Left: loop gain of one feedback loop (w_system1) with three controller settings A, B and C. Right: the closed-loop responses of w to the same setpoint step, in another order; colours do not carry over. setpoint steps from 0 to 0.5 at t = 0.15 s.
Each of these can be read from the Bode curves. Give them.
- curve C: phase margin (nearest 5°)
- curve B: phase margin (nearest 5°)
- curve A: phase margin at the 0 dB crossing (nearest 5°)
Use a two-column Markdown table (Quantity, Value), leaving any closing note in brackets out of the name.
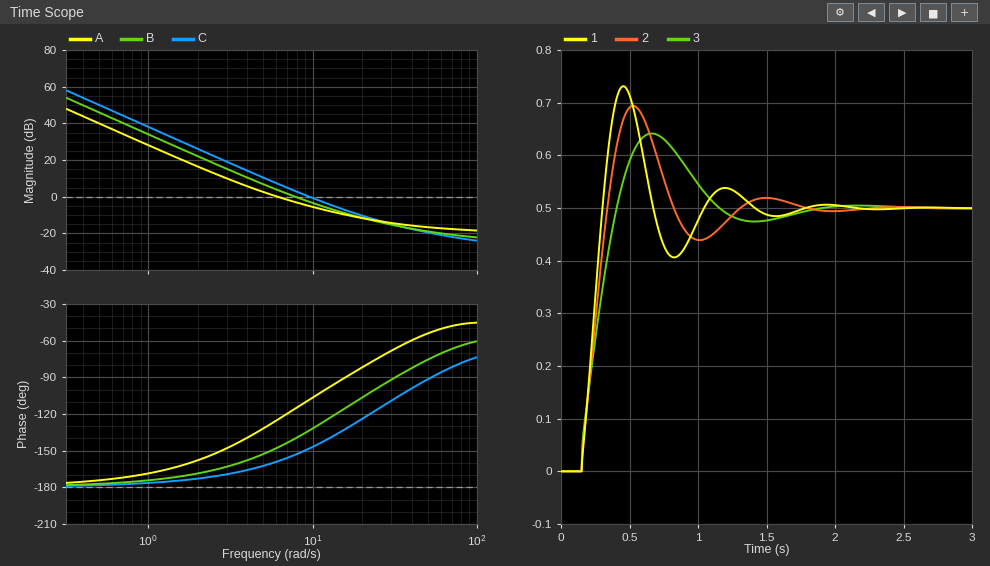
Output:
| Quantity | Value |
|---|---|
| curve C: phase margin | 30° |
| curve B: phase margin | 40° |
| curve A: phase margin at the 0 dB crossing | 55° |
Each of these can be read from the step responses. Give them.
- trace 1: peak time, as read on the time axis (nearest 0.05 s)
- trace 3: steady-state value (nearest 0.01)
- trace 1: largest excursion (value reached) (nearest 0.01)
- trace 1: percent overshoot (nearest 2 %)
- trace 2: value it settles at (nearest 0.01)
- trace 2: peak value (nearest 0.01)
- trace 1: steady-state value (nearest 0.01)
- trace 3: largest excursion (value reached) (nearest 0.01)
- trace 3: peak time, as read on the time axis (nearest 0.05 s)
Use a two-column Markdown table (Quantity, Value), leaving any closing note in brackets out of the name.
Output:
| Quantity | Value |
|---|---|
| trace 1: peak time, as read on the time axis | 0.45 s |
| trace 3: steady-state value | 0.50 |
| trace 1: largest excursion (value reached) | 0.73 |
| trace 1: percent overshoot | 46 % |
| trace 2: value it settles at | 0.50 |
| trace 2: peak value | 0.69 |
| trace 1: steady-state value | 0.50 |
| trace 3: largest excursion (value reached) | 0.64 |
| trace 3: peak time, as read on the time axis | 0.65 s |
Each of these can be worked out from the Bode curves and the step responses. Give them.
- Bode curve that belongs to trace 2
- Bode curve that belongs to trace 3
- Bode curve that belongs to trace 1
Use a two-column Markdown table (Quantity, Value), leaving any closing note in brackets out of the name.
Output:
| Quantity | Value |
|---|---|
| Bode curve that belongs to trace 2 | B |
| Bode curve that belongs to trace 3 | A |
| Bode curve that belongs to trace 1 | C |
